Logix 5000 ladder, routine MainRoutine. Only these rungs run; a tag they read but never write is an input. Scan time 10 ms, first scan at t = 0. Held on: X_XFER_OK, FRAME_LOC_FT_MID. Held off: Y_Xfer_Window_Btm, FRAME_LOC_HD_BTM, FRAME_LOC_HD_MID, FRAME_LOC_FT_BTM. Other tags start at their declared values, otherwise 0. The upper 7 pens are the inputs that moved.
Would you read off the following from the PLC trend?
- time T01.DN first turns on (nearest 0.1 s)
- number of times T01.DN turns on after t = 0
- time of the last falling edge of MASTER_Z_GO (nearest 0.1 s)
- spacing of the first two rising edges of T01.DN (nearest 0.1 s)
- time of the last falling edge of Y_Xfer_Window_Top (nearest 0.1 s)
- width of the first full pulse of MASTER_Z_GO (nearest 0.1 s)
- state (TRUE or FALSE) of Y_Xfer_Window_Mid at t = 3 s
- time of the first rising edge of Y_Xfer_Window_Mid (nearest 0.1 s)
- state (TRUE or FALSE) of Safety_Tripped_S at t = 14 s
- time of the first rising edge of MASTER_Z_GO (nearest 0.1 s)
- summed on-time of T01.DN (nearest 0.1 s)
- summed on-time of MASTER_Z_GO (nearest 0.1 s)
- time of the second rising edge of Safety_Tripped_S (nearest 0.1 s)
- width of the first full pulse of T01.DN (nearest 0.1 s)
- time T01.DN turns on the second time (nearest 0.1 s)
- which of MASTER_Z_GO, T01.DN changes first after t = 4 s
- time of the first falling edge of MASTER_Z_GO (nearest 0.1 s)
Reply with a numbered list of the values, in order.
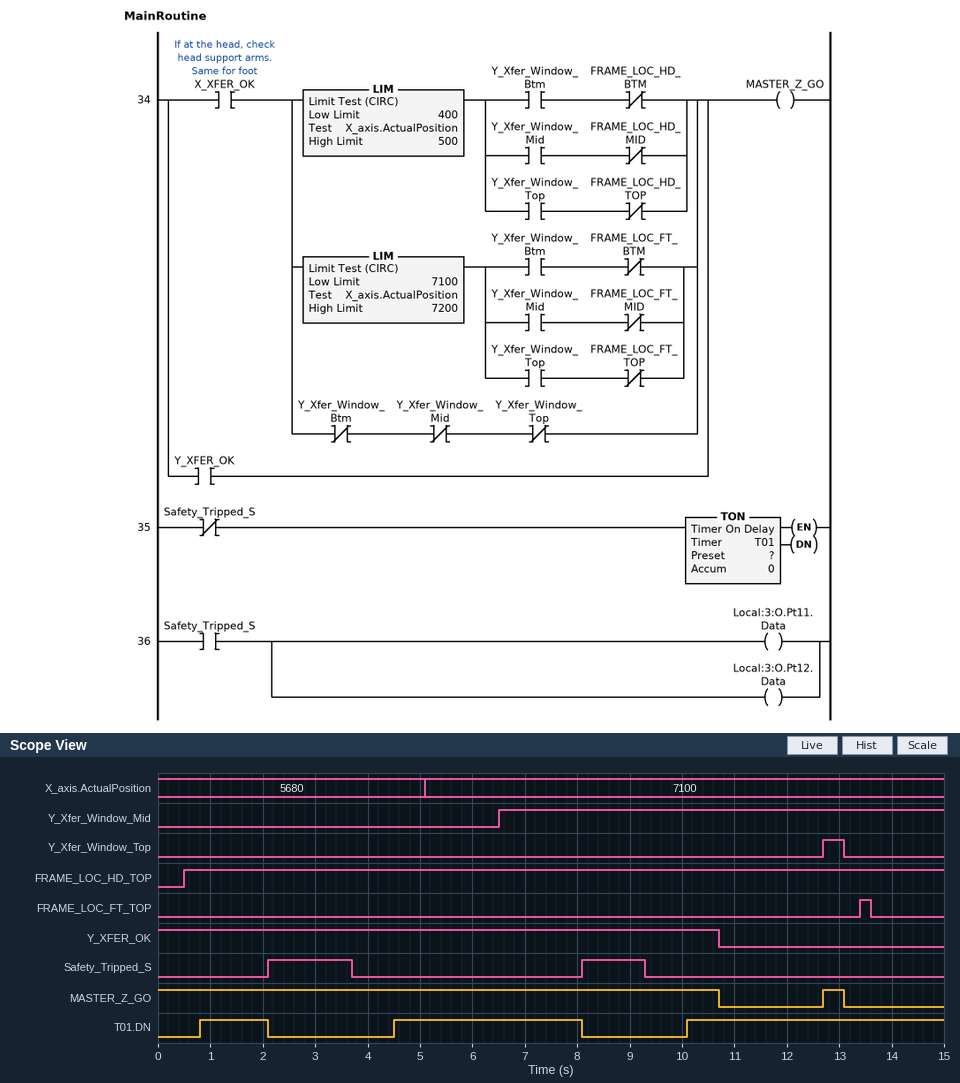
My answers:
1. 0.8 s
2. 3
3. 13.1 s
4. 3.7 s
5. 13.1 s
6. 0.4 s
7. FALSE
8. 6.5 s
9. FALSE
10. 12.7 s
11. 9.8 s
12. 11.1 s
13. 8.1 s
14. 1.3 s
15. 4.5 s
16. T01.DN
17. 10.7 s
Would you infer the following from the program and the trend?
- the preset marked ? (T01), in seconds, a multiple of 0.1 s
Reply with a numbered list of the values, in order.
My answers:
1. 0.8 s
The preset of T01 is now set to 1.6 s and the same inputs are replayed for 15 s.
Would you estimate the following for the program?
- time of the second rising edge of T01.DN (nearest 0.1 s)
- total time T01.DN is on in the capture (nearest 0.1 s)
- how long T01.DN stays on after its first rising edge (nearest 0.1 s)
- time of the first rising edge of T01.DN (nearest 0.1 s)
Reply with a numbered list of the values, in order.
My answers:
1. 5.3 s
2. 7.4 s
3. 0.5 s
4. 1.6 s
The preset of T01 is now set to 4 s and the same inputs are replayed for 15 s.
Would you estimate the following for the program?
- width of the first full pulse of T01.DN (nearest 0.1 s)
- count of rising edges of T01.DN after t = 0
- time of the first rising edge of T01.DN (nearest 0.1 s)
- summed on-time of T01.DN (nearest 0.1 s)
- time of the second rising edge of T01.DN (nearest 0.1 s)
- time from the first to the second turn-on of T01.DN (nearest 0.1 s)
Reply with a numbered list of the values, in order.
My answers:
1. 0.4 s
2. 2
3. 7.7 s
4. 2.1 s
5. 13.3 s
6. 5.6 s
